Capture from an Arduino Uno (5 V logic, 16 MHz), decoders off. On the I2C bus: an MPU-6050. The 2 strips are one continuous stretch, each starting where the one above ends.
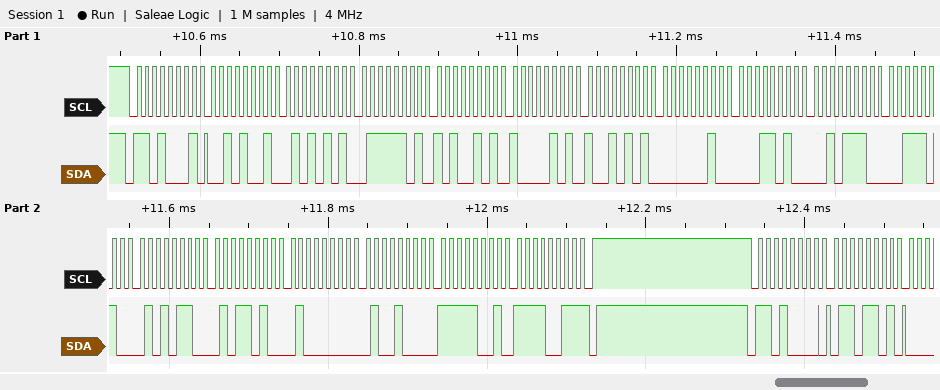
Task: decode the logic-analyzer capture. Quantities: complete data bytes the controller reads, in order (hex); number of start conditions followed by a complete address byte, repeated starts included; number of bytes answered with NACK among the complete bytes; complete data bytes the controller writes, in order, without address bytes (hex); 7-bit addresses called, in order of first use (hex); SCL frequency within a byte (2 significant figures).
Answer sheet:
29 55 7D A5 85 95 02 1A 2E 3A 56 5A 40 48 F9 F3
2
1
6D
0x68
100 kHz
